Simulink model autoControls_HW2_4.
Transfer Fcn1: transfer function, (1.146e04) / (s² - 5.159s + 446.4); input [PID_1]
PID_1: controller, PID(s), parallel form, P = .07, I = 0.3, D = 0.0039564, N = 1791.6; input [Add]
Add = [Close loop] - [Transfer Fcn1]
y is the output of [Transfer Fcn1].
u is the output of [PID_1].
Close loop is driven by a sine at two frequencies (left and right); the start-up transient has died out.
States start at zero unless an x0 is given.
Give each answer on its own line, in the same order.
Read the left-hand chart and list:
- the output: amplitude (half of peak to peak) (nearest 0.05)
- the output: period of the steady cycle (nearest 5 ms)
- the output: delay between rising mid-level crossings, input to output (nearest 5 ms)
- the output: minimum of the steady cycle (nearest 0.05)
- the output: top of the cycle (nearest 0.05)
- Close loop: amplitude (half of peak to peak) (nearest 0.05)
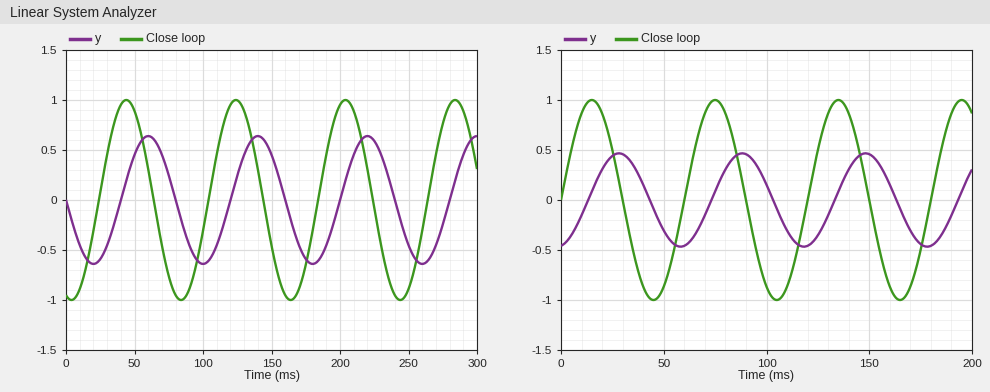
0.65
80 ms
15 ms
-0.65
0.65
1.00
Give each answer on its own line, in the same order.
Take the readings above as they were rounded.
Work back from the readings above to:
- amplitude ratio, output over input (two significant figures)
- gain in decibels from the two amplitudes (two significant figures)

0.65
-3.7 dB
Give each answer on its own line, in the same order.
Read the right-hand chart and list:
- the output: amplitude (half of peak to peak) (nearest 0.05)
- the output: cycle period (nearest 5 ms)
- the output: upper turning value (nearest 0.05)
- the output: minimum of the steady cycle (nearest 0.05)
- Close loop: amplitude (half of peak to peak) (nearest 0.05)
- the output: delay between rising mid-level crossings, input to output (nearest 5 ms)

0.45
60 ms
0.45
-0.45
1.00
15 ms
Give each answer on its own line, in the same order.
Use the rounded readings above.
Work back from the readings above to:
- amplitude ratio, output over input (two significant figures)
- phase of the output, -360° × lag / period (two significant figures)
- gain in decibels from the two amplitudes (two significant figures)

0.45
-90°
-6.9 dB
